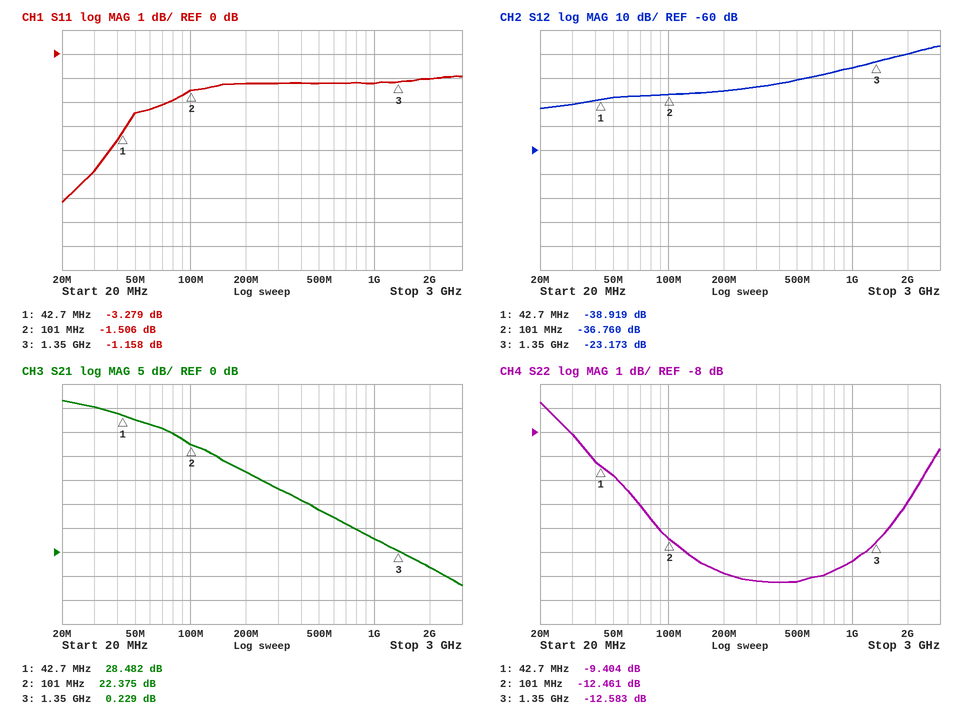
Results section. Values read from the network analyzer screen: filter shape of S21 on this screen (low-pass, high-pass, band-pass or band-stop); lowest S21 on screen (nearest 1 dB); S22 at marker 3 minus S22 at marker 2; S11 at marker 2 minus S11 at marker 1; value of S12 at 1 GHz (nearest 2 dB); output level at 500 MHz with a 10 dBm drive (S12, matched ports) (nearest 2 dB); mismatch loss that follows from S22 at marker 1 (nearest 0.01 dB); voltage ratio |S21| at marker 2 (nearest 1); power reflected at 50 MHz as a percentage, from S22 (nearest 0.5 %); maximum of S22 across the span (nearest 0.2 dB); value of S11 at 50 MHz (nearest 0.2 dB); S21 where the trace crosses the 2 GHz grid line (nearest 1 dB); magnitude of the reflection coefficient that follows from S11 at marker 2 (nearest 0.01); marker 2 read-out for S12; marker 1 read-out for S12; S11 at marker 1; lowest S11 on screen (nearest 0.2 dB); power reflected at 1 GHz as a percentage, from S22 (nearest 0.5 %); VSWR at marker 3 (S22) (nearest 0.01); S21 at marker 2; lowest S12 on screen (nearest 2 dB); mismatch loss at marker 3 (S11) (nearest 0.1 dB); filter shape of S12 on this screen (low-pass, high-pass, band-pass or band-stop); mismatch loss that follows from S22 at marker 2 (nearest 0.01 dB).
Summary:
low-pass
-7 dB
-0.122 dB
1.773 dB
-26 dB
-20 dBm
0.53 dB
13
10.5 %
-6.8 dB
-2.4 dB
-3 dB
0.84
-36.760 dB
-38.919 dB
-3.279 dB
-6.2 dB
4.5 %
1.61
22.375 dB
-42 dB
6.3 dB
high-pass
0.25 dB
